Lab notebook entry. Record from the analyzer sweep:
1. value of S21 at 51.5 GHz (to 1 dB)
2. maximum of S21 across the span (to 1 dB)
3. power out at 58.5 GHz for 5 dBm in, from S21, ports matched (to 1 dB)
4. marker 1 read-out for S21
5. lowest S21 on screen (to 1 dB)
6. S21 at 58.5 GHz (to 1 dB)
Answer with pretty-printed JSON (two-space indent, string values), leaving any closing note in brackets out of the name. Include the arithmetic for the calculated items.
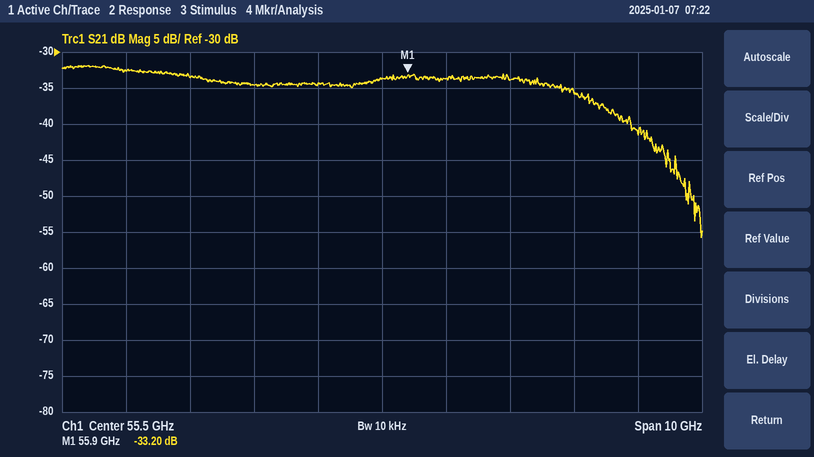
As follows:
{
  "value of S21 at 51.5 GHz": "-33 dB",
  "maximum of S21 across the span": "-32 dB",
  "power out at 58.5 GHz for 5 dBm in, from S21, ports matched": "5 dBm + (-36 dB) = -31 dBm",
  "marker 1 read-out for S21": "-33.20 dB",
  "lowest S21 on screen": "-56 dB",
  "S21 at 58.5 GHz": "-36 dB"
}
